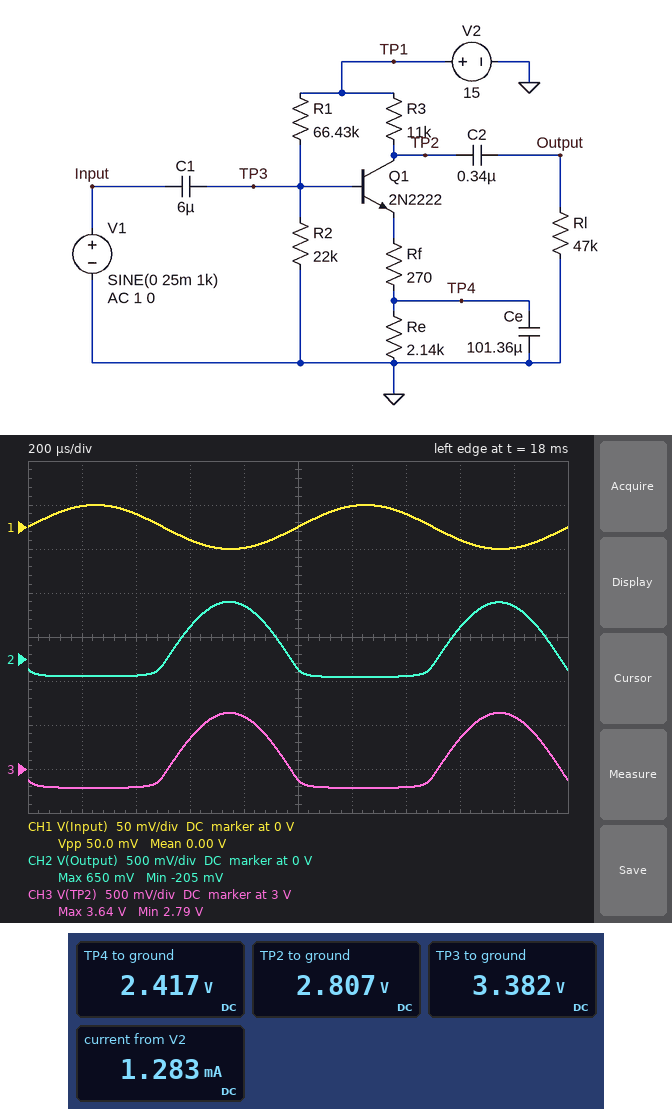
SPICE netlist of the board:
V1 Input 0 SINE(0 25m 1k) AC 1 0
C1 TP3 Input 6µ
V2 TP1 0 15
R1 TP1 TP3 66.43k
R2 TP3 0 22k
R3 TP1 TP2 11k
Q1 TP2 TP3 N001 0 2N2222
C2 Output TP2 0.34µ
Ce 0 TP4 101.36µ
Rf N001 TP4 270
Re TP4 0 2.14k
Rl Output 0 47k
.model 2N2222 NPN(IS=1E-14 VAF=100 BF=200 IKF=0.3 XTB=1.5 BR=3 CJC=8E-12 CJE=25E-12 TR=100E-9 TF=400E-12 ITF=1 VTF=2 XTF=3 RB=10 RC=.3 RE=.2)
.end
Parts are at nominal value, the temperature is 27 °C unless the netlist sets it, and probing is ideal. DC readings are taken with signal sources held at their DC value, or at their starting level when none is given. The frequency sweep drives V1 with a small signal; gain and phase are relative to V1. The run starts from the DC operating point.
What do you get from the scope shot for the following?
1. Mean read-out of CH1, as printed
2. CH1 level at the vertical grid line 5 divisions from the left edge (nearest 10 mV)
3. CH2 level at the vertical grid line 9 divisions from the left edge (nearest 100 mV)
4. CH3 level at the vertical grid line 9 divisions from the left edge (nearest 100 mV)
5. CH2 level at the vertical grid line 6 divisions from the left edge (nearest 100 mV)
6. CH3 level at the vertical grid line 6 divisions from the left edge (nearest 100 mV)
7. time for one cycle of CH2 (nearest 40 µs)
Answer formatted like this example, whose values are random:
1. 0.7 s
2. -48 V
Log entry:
1. 0.00 V
2. 0 V
3. 600 mV
4. 3.6 V
5. -200 mV
6. 2.8 V
7. 1.00 ms
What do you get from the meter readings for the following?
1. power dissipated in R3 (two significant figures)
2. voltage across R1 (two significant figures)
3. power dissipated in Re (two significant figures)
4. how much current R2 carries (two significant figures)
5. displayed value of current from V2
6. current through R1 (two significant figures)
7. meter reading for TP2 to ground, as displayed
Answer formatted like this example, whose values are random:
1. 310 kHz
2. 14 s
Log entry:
1. 14 mW
2. 12 V
3. 2.7 mW
4. 150 µA
5. 1.283 mA
6. 170 µA
7. 2.807 V
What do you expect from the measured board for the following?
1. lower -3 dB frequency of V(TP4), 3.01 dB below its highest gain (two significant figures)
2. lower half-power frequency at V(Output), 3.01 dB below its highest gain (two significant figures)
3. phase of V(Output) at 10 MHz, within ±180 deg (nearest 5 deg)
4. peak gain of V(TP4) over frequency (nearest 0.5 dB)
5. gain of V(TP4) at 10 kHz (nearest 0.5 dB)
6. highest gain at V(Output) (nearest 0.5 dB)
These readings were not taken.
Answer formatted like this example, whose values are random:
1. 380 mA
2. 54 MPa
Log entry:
1. 910 mHz
2. 72 Hz
3. 15 deg
4. -24.5 dB
5. -67.0 dB
6. 10.0 dB
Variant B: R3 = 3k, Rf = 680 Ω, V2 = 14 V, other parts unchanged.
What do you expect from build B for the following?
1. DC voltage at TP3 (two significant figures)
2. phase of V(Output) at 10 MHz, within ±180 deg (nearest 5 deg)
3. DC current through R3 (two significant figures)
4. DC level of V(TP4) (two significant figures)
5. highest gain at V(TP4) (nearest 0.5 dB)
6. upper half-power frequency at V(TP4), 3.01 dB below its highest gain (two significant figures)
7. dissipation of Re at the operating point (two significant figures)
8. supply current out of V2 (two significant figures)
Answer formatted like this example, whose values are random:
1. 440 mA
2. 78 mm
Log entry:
1. 3.4 V
2. 135 deg
3. 970 µA
4. 2.1 V
5. -6.5 dB
6. 5.6 Hz
7. 2.0 mW
8. 1.1 mA
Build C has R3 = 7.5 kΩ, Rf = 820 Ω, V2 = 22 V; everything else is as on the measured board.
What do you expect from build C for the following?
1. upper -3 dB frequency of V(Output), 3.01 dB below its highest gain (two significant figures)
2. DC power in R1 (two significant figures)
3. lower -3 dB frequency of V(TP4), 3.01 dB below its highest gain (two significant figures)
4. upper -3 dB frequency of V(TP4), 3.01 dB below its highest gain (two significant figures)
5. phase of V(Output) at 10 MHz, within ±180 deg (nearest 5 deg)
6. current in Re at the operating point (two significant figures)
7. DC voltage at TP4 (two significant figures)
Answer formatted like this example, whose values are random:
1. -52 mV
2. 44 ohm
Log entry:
1. 6.0 MHz
2. 4.2 mW
3. 830 mHz
4. 5.2 Hz
5. 105 deg
6. 1.6 mA
7. 3.4 V
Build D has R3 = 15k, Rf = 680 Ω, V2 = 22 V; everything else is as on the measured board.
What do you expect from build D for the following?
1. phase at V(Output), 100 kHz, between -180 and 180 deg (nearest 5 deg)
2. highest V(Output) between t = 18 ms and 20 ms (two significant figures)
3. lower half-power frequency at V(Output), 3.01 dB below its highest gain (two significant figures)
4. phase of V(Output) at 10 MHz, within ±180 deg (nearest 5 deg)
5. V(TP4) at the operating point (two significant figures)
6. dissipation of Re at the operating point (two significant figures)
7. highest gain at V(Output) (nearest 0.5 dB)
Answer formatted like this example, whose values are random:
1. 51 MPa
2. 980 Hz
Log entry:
1. 10 deg
2. 12 mV
3. 450 kHz
4. 0 deg
5. 2.8 V
6. 3.6 mW
7. 0 dB
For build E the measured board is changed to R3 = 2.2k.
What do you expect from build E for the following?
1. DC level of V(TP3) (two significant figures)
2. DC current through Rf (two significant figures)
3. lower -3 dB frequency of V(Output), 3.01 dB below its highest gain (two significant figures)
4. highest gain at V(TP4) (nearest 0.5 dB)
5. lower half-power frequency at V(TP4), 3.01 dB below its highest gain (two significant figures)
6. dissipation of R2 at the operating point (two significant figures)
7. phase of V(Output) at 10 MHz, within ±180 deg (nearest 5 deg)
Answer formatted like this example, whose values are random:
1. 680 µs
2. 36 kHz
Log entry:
1. 3.6 V
2. 1.2 mA
3. 13 Hz
4. -3.5 dB
5. 1.1 Hz
6. 600 µW
7. 145 deg
